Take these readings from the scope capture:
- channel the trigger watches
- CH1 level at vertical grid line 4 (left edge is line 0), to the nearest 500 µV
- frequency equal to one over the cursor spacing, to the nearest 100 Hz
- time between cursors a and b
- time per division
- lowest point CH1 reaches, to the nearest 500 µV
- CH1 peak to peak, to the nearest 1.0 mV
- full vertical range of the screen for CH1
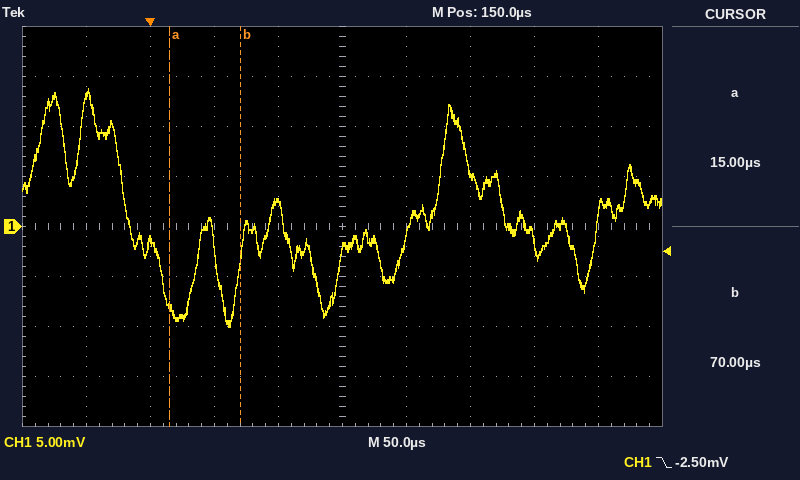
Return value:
CH1
2.5 mV
18.2 kHz
55 µs
50 µs
-10.0 mV
24.0 mV
40 mV
